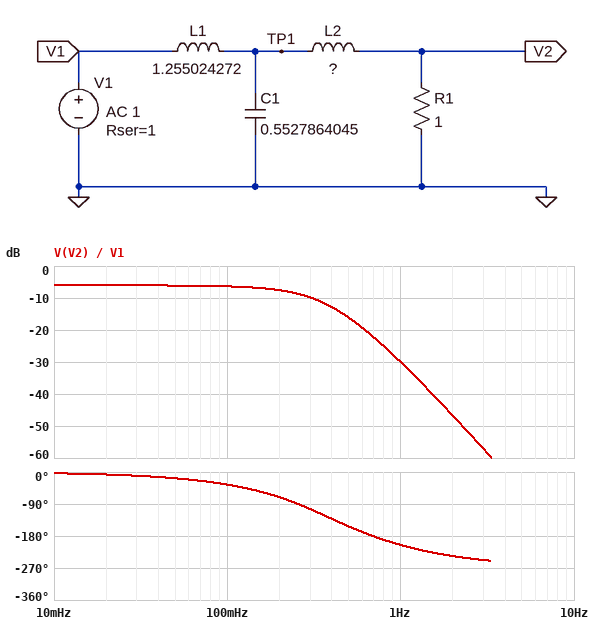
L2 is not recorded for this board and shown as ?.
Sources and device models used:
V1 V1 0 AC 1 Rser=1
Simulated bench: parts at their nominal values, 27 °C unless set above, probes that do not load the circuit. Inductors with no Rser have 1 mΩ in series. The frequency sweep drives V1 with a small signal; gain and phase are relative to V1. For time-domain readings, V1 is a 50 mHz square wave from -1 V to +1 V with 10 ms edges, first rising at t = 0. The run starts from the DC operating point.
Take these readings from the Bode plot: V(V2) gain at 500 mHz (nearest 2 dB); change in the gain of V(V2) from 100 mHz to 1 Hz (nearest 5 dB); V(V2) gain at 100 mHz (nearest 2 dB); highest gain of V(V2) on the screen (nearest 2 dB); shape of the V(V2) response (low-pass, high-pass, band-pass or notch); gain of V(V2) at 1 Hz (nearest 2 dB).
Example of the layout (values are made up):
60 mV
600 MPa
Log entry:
-16 dB
-25 dB
-6 dB
-6 dB
low-pass
-30 dB
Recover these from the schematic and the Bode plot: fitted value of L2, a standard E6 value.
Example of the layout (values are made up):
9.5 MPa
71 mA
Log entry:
150 mH
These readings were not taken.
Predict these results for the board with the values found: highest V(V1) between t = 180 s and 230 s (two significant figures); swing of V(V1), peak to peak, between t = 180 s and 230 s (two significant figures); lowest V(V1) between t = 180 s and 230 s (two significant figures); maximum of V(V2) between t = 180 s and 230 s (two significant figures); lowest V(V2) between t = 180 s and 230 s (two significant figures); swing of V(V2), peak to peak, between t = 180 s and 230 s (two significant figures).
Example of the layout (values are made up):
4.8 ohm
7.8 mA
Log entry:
1.5 V
3.0 V
-1.5 V
510 mV
-510 mV
1.0 V
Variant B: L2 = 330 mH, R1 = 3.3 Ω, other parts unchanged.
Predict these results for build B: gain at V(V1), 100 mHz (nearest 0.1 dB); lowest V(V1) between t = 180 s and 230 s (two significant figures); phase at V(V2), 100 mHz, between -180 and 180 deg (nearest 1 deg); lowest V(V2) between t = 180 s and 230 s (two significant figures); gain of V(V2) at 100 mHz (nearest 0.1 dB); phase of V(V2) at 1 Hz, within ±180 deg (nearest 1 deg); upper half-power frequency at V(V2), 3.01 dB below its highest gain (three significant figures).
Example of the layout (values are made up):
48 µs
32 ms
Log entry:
-3.7 dB
-1.2 V
-32 deg
-1.0 V
-1.5 dB
159 deg
262 mHz
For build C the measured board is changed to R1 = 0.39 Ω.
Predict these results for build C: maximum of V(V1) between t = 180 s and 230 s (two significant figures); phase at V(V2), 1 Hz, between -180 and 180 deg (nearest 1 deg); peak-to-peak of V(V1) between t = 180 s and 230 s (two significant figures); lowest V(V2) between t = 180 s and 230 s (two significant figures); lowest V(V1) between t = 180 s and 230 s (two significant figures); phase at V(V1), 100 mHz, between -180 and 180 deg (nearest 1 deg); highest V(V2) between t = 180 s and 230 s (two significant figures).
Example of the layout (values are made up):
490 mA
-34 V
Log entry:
1.7 V
129 deg
3.4 V
-280 mV
-1.7 V
33 deg
280 mV
